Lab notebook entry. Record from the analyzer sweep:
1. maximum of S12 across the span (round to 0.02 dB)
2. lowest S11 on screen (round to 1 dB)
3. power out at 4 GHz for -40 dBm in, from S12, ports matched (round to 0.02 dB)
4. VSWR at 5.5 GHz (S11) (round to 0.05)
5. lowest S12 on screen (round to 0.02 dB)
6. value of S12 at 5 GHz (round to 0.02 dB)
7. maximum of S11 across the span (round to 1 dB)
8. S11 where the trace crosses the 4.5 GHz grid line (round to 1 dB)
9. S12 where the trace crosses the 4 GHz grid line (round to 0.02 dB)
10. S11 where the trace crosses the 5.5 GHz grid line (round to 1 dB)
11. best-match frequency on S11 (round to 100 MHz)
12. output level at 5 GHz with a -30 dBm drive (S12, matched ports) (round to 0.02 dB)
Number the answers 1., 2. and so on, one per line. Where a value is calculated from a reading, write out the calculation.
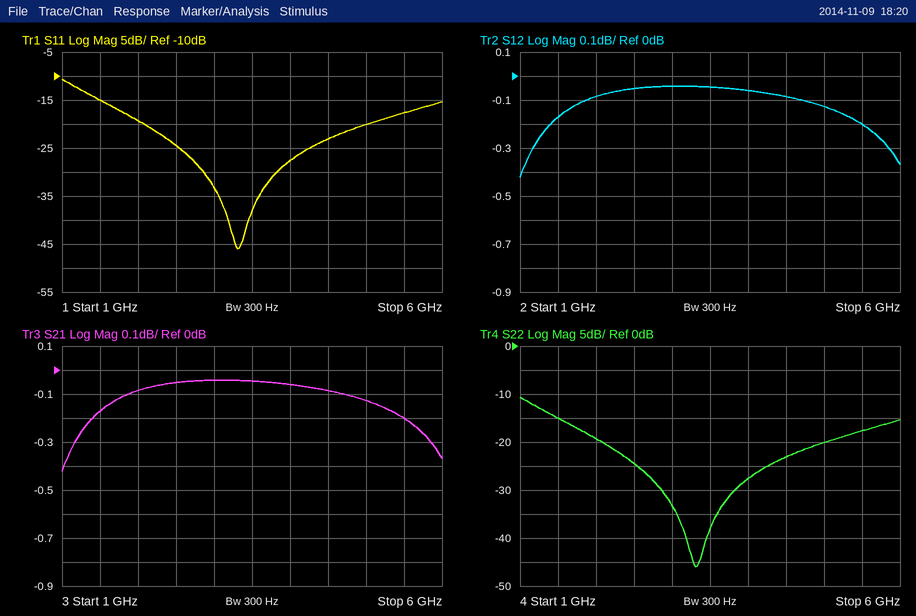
1. -0.04 dB
2. -46 dB
3. -40 dBm + (-0.06 dB) = -40.06 dBm
4. |Γ| = 10^(-18/20) = 0.1259; VSWR = (1 + 0.1259)/(1 − 0.1259) ≈ 1.29, so 1.30 to the nearest 0.05
5. -0.42 dB
6. -0.12 dB
7. -11 dB
8. -23 dB
9. -0.06 dB
10. -18 dB
11. 3.3 GHz
12. -30 dBm + (-0.12 dB) = -30.12 dBm
